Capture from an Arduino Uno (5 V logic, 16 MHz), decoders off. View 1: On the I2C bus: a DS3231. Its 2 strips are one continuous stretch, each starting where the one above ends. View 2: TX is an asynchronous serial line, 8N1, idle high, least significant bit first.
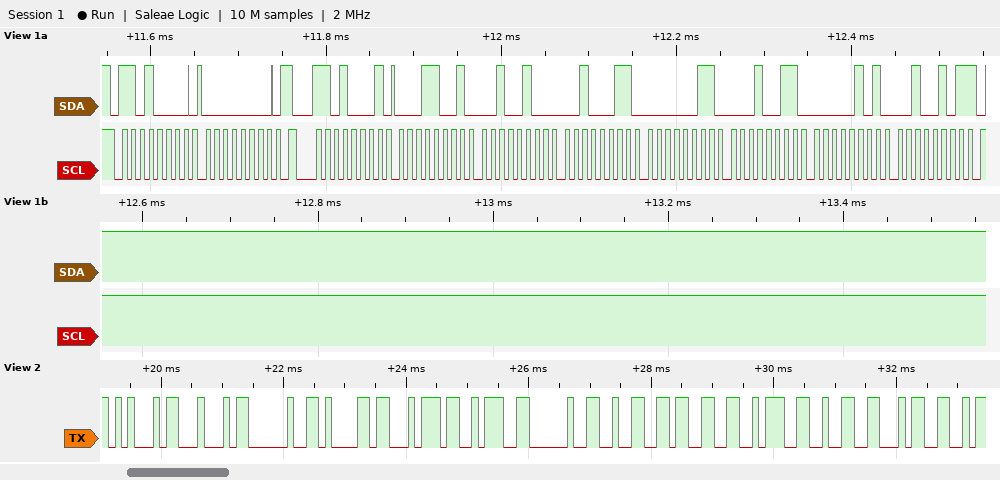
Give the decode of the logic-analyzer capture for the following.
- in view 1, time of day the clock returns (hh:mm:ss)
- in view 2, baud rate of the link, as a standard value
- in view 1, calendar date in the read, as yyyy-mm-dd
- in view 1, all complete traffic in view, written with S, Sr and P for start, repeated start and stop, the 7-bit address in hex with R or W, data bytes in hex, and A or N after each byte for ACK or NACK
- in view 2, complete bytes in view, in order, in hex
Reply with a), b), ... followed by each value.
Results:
a) 23:24:19
b) 9600 baud
c) 2025-05-13
d) S 68W A 00 A Sr 68R A 19 A 24 A 23 A 03 A 13 A 05 A 25 N P
e) 45 44 20 61 74 3A 20 32 33 3A 32 34
